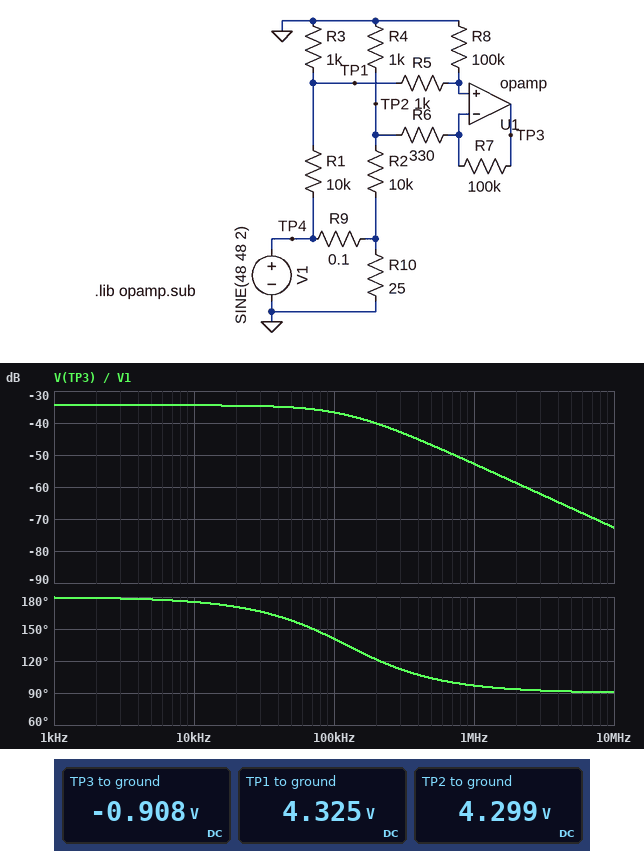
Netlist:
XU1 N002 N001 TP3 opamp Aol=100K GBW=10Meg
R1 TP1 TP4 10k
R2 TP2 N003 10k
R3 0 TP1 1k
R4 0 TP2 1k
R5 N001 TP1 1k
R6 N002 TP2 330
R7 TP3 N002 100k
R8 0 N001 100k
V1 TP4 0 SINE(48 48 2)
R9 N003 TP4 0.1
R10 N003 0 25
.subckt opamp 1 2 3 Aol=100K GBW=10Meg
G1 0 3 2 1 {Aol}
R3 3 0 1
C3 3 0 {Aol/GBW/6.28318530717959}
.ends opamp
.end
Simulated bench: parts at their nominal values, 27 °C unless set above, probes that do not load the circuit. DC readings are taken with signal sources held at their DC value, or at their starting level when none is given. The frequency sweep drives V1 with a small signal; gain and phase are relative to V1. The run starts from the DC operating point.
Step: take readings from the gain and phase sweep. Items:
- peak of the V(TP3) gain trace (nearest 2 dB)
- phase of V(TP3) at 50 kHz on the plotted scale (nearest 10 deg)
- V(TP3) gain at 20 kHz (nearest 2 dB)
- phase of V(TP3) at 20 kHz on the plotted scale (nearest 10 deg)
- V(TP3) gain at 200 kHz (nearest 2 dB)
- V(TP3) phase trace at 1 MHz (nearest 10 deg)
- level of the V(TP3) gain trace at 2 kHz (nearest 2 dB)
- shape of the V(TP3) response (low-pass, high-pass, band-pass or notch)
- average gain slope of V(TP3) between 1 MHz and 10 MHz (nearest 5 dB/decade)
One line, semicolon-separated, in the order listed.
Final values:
-34 dB; 160 deg; -34 dB; 170 deg; -40 dB; 100 deg; -34 dB; low-pass; -20 dB/decade
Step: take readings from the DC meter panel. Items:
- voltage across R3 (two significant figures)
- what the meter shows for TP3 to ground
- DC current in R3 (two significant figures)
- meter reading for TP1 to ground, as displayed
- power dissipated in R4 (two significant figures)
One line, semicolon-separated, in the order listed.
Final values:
4.3 V; -0.908 V; 4.3 mA; 4.325 V; 18 mW
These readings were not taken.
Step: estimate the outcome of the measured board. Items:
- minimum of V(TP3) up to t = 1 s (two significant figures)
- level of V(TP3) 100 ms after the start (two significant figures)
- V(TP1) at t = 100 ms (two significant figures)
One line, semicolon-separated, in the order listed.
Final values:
-1.8 V; -1.8 V; 8.4 V
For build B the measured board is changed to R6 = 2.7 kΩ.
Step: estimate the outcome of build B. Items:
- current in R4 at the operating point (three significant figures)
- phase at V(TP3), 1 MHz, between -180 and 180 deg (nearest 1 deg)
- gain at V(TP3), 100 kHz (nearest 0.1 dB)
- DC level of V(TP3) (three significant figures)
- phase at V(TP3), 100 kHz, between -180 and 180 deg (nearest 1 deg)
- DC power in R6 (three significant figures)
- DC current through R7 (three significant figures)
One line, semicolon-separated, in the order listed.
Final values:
4.33 mA; -71 deg; -26.0 dB; 2.50 V; -16 deg; 858 nW; 17.8 µA
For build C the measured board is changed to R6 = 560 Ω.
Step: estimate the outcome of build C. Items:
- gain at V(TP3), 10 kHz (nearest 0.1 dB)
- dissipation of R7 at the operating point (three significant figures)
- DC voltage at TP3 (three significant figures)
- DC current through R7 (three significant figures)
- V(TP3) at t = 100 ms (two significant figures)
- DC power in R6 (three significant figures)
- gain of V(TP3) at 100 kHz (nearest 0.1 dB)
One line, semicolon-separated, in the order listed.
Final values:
-54.0 dB; 192 µW; -96.3 mV; 43.8 µA; -190 mV; 1.07 µW; -55.6 dB
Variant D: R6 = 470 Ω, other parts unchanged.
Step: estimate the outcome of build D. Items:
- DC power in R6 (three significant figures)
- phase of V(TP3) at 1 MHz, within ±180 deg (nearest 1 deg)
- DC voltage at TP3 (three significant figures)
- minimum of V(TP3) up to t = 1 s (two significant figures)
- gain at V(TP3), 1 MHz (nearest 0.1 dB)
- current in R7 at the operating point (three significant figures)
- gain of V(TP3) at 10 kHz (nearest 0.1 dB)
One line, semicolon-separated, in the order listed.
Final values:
1.02 µW; 98 deg; -382 mV; -760 mV; -59.4 dB; 46.6 µA; -42.0 dB
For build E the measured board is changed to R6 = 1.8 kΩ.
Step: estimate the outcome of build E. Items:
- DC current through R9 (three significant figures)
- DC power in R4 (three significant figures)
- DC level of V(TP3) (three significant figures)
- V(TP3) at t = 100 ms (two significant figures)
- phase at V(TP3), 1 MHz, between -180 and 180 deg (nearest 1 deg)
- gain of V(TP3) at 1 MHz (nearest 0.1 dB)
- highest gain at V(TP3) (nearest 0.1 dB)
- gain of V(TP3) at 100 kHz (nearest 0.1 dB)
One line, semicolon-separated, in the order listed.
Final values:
1.92 A; 18.7 mW; 1.91 V; 3.7 V; -75 deg; -39.9 dB; -28.0 dB; -28.6 dB
